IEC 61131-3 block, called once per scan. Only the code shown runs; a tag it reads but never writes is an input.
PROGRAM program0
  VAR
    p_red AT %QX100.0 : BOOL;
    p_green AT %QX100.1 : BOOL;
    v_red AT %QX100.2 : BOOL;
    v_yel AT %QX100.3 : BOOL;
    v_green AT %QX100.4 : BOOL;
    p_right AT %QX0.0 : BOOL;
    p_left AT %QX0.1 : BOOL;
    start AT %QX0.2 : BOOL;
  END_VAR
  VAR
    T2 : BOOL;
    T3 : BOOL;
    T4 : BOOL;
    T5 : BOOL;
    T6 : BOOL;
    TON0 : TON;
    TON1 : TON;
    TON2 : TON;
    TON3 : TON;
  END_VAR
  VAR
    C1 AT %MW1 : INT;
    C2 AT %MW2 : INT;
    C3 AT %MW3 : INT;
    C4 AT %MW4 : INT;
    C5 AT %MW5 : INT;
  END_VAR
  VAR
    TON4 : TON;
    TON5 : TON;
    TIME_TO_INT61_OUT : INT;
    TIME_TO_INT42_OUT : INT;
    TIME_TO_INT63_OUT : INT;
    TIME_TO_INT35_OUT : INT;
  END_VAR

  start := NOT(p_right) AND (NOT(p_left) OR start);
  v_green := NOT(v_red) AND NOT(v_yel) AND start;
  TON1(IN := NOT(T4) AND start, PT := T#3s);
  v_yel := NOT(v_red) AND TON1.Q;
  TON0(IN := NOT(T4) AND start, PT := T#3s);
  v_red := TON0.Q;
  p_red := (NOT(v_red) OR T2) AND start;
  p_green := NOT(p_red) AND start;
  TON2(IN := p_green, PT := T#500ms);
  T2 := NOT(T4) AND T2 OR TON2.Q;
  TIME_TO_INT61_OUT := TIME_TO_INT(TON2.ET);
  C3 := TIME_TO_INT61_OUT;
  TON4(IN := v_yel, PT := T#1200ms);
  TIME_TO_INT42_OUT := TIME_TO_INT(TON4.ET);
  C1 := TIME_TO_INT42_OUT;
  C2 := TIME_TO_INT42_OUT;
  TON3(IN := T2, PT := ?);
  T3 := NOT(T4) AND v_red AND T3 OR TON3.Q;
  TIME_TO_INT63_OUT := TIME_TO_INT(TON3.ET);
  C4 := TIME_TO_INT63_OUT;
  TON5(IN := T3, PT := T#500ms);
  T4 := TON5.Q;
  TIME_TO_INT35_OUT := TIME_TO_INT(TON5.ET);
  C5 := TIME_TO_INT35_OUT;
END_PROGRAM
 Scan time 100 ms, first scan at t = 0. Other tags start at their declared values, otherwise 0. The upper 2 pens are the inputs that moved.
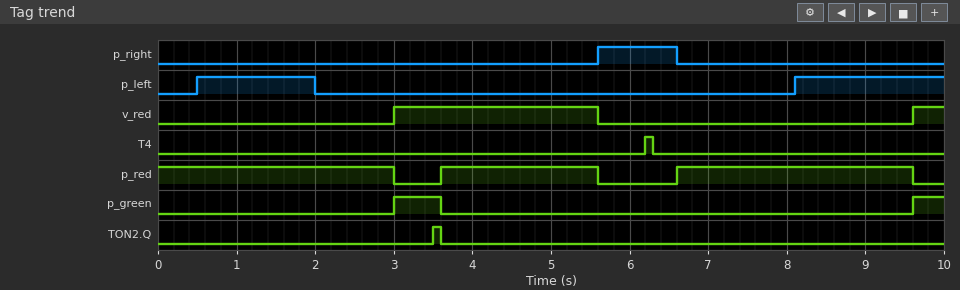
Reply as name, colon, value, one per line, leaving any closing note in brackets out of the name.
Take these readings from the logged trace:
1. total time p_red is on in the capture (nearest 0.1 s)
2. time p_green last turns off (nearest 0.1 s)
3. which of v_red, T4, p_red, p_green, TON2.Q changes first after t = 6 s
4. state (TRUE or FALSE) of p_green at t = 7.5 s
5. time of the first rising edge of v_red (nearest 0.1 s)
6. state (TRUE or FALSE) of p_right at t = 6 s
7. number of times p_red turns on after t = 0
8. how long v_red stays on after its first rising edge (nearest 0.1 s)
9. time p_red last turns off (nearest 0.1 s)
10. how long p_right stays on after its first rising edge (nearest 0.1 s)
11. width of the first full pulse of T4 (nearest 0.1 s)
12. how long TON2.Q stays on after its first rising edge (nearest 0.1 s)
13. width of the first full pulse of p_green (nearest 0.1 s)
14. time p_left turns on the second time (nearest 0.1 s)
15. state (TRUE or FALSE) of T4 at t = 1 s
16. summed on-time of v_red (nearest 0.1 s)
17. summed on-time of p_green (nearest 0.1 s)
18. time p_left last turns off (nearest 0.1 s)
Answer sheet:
total time p_red is on in the capture: 8.0 s
time p_green last turns off: 3.6 s
which of v_red, T4, p_red, p_green, TON2.Q changes first after t = 6 s: T4
state (TRUE or FALSE) of p_green at t = 7.5 s: FALSE
time of the first rising edge of v_red: 3.0 s
state (TRUE or FALSE) of p_right at t = 6 s: TRUE
number of times p_red turns on after t = 0: 2
how long v_red stays on after its first rising edge: 2.6 s
time p_red last turns off: 9.6 s
how long p_right stays on after its first rising edge: 1.0 s
width of the first full pulse of T4: 0.1 s
how long TON2.Q stays on after its first rising edge: 0.1 s
width of the first full pulse of p_green: 0.6 s
time p_left turns on the second time: 8.1 s
state (TRUE or FALSE) of T4 at t = 1 s: FALSE
summed on-time of v_red: 3.0 s
summed on-time of p_green: 1.0 s
time p_left last turns off: 2.0 s
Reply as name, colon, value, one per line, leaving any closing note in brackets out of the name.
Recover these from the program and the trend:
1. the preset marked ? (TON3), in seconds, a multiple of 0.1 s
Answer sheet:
the preset marked ? (TON3), in seconds, a multiple of 0.1 s: 2.2 s
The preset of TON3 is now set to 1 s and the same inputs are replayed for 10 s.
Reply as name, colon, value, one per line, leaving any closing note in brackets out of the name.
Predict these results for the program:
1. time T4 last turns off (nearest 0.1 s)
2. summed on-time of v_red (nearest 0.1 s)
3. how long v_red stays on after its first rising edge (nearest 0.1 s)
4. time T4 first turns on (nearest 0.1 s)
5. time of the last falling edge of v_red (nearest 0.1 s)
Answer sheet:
time T4 last turns off: 5.1 s
summed on-time of v_red: 2.5 s
how long v_red stays on after its first rising edge: 2.1 s
time T4 first turns on: 5.0 s
time of the last falling edge of v_red: 5.1 s
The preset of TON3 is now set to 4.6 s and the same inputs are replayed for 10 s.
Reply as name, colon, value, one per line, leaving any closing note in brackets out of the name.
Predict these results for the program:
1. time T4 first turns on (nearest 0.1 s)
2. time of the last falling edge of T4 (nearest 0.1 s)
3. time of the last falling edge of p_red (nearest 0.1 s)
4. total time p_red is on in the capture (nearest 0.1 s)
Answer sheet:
time T4 first turns on: 8.6 s
time of the last falling edge of T4: 8.7 s
time of the last falling edge of p_red: 5.6 s
total time p_red is on in the capture: 8.4 s
